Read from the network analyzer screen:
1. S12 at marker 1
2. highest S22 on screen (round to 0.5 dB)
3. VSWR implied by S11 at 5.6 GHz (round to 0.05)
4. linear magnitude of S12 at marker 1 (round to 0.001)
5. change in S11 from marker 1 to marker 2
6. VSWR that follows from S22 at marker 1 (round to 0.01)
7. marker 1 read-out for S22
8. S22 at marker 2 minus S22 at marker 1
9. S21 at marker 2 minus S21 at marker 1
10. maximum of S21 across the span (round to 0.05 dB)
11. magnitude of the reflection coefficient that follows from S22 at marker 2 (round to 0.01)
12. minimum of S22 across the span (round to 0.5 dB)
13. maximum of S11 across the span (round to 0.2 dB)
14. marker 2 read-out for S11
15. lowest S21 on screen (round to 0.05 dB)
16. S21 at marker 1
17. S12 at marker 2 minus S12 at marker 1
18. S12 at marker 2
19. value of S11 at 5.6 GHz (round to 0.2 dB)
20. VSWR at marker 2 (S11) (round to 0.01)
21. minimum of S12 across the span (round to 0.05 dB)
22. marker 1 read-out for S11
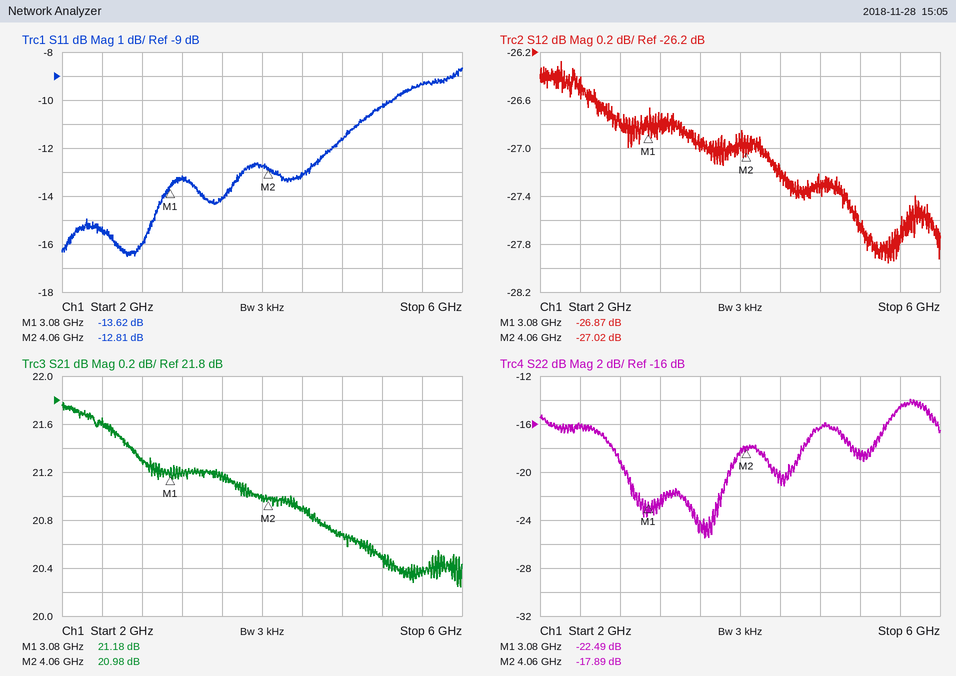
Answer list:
-26.87 dB
-14.0 dB
2.05
0.045
0.81 dB
1.16
-22.49 dB
4.60 dB
-0.20 dB
21.80 dB
0.13
-25.5 dB
-8.6 dB
-12.81 dB
20.25 dB
21.18 dB
-0.15 dB
-27.02 dB
-9.4 dB
1.59
-27.95 dB
-13.62 dB
